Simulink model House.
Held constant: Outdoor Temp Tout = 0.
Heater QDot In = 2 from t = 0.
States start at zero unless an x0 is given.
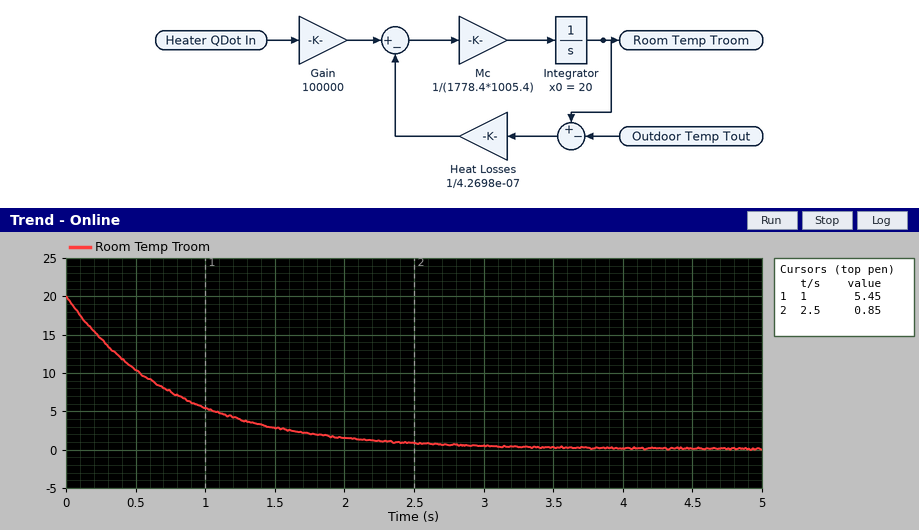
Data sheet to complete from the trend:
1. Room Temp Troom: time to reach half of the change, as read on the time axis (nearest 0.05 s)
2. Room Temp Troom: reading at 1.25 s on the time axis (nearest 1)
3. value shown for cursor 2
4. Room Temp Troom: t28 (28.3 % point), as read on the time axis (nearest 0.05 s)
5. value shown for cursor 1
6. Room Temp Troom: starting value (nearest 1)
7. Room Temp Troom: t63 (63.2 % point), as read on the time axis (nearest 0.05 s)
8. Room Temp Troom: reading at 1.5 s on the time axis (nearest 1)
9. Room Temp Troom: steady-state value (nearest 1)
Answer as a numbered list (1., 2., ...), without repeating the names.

1. 0.55 s
2. 4
3. 0.85
4. 0.25 s
5. 5.45
6. 20
7. 0.75 s
8. 3
9. 0
